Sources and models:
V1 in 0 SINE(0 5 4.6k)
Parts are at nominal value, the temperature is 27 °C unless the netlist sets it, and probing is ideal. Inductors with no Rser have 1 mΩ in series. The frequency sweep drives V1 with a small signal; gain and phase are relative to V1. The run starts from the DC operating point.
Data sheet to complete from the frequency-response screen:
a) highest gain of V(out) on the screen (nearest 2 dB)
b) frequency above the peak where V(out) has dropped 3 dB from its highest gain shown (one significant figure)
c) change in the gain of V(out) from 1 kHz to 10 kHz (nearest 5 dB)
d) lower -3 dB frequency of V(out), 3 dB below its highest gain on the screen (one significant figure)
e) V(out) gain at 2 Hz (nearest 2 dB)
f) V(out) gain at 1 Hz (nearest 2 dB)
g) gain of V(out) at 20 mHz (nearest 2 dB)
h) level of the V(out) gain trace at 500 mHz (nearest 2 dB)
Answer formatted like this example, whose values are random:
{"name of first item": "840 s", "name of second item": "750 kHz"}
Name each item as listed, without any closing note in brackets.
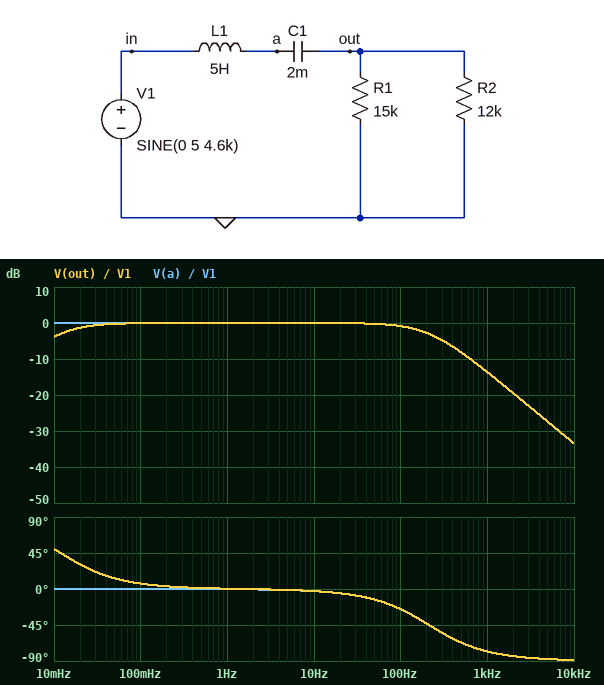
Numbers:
{"highest gain of V(out) on the screen": "0 dB", "frequency above the peak where V(out) has dropped 3 dB from its highest gain shown": "200 Hz", "change in the gain of V(out) from 1 kHz to 10 kHz": "-20 dB", "lower -3 dB frequency of V(out), 3 dB below its highest gain on the screen": "10 mHz", "V(out) gain at 2 Hz": "0 dB", "V(out) gain at 1 Hz": "0 dB", "gain of V(out) at 20 mHz": "-2 dB", "level of the V(out) gain trace at 500 mHz": "0 dB"}
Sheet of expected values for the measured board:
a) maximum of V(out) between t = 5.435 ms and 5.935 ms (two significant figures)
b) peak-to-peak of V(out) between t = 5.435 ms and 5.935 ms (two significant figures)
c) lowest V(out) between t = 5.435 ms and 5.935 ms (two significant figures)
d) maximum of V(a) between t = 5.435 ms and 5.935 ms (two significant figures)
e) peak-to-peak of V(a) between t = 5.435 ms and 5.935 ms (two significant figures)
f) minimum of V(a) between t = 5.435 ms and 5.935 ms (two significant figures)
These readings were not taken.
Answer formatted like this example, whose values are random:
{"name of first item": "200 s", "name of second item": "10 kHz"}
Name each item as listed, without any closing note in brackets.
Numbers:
{"maximum of V(out) between t = 5.435 ms and 5.935 ms": "230 mV", "peak-to-peak of V(out) between t = 5.435 ms and 5.935 ms": "460 mV", "lowest V(out) between t = 5.435 ms and 5.935 ms": "-230 mV", "maximum of V(a) between t = 5.435 ms and 5.935 ms": "230 mV", "peak-to-peak of V(a) between t = 5.435 ms and 5.935 ms": "460 mV", "minimum of V(a) between t = 5.435 ms and 5.935 ms": "-230 mV"}
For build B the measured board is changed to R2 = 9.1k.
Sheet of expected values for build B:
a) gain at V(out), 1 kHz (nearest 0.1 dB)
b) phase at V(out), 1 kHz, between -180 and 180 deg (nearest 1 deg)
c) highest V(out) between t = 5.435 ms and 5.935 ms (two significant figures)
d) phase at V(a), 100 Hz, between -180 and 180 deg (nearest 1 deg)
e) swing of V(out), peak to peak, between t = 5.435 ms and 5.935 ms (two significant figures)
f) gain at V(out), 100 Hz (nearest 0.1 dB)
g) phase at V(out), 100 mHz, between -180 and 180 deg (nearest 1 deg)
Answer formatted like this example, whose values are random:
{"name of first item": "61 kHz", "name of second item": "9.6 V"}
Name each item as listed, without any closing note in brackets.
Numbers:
{"gain at V(out), 1 kHz": "-15.0 dB", "phase at V(out), 1 kHz, between -180 and 180 deg": "-80 deg", "highest V(out) between t = 5.435 ms and 5.935 ms": "200 mV", "phase at V(a), 100 Hz, between -180 and 180 deg": "-29 deg", "swing of V(out), peak to peak, between t = 5.435 ms and 5.935 ms": "390 mV", "gain at V(out), 100 Hz": "-1.2 dB", "phase at V(out), 100 mHz, between -180 and 180 deg": "8 deg"}
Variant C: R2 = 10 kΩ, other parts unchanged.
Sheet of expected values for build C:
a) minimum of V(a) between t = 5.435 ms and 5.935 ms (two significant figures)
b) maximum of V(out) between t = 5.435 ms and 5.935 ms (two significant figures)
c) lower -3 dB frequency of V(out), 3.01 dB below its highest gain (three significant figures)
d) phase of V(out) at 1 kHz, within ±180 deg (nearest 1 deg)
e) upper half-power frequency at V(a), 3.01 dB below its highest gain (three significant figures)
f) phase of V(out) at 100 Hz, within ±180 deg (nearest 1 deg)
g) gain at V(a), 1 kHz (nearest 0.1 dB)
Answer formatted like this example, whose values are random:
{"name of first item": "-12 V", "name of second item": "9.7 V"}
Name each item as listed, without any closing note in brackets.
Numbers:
{"minimum of V(a) between t = 5.435 ms and 5.935 ms": "-210 mV", "maximum of V(out) between t = 5.435 ms and 5.935 ms": "210 mV", "lower -3 dB frequency of V(out), 3.01 dB below its highest gain": "13.3 mHz", "phase of V(out) at 1 kHz, within ±180 deg": "-79 deg", "upper half-power frequency at V(a), 3.01 dB below its highest gain": "191 Hz", "phase of V(out) at 100 Hz, within ±180 deg": "-28 deg", "gain at V(a), 1 kHz": "-14.5 dB"}
